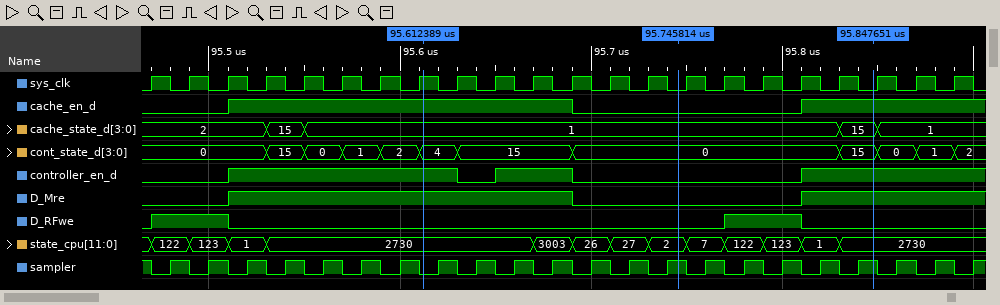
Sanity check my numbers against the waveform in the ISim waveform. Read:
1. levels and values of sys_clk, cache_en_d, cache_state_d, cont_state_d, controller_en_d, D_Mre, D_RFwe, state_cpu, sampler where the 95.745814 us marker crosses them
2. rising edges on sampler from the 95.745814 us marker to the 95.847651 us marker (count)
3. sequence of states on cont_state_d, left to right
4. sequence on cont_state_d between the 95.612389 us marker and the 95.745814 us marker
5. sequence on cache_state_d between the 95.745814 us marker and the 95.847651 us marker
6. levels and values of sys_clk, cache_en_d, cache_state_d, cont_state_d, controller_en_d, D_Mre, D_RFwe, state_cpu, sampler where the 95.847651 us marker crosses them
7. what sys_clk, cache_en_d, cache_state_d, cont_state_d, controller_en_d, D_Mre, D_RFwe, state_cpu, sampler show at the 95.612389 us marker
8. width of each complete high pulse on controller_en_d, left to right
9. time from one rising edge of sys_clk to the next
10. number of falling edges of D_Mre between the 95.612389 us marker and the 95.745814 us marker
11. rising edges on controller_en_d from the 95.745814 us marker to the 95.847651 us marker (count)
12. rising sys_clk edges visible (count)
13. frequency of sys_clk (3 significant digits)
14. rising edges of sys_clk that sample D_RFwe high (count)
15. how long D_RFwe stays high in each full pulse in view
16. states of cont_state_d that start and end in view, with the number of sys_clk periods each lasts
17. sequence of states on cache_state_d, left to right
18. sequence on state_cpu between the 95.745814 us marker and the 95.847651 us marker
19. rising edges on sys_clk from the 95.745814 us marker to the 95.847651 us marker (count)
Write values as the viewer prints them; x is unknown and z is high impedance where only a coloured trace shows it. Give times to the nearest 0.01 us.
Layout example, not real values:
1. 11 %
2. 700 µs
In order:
1. sys_clk=0, cache_en_d=0, cache_state_d=1, cont_state_d=0, controller_en_d=0, D_Mre=0, D_RFwe=0, state_cpu=2, sampler=1
2. 5
3. 0, 15, 0, 1, 2, 4, 15, 0, 15, 0, 1, 2
4. 4, 15, 0
5. 1, 15
6. sys_clk=0, cache_en_d=1, cache_state_d=15, cont_state_d=15, controller_en_d=1, D_Mre=1, D_RFwe=0, state_cpu=2730, sampler=1
7. sys_clk=1, cache_en_d=1, cache_state_d=1, cont_state_d=4, controller_en_d=1, D_Mre=1, D_RFwe=0, state_cpu=2730, sampler=0
8. 0.12 us, 0.04 us
9. 0.02 us
10. 1
11. 1
12. 22
13. 50.0 MHz
14. 4
15. 0.04 us, 0.04 us
16. 15: 1, 0: 1, 1: 1, 2: 1, 4: 1, 15: 3, 0: 7, 15: 1, 0: 1, 1: 1
17. 2, 15, 1, 15, 1
18. 2, 7, 122, 123, 1, 2730
19. 5
